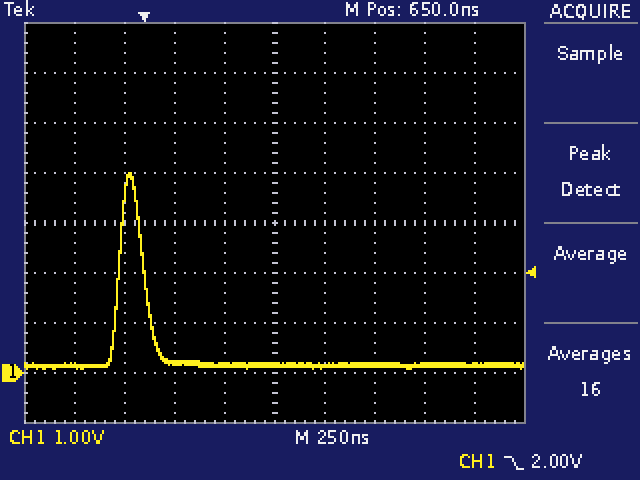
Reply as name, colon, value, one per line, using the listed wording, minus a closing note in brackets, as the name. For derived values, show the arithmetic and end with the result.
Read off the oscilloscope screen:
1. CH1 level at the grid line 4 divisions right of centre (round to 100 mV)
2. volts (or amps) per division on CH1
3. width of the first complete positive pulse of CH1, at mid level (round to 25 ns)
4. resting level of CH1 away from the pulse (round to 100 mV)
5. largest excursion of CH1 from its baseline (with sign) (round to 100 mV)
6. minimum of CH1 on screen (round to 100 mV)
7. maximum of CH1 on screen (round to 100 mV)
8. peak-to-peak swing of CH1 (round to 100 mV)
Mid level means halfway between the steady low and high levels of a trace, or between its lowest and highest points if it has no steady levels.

CH1 level at the grid line 4 divisions right of centre: 200 mV
volts (or amps) per division on CH1: 1 V
width of the first complete positive pulse of CH1, at mid level: 125 ns
resting level of CH1 away from the pulse: 200 mV
largest excursion of CH1 from its baseline (with sign): 4.0 V − (200 mV) = +3.8 V
minimum of CH1 on screen: 100 mV
maximum of CH1 on screen: 4.0 V
peak-to-peak swing of CH1: 4.0 V − (100 mV) = 3.9 V
